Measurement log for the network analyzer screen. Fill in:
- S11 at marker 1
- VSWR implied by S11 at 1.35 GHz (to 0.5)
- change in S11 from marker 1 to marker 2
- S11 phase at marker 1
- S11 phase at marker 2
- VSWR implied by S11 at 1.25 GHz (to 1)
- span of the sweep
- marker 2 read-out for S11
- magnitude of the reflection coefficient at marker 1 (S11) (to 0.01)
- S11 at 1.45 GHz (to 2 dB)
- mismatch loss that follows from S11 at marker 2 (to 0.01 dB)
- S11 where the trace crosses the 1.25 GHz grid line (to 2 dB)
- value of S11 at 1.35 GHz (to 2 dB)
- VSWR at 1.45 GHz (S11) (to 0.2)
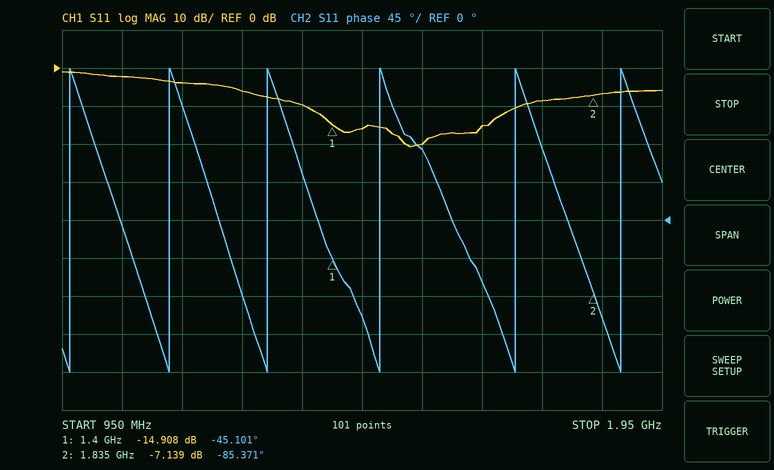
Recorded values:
-14.908 dB
2.0
7.769 dB
-45.101°
-85.371°
3
1 GHz
-7.139 dB
0.18
-16 dB
0.93 dB
-6 dB
-10 dB
1.4
